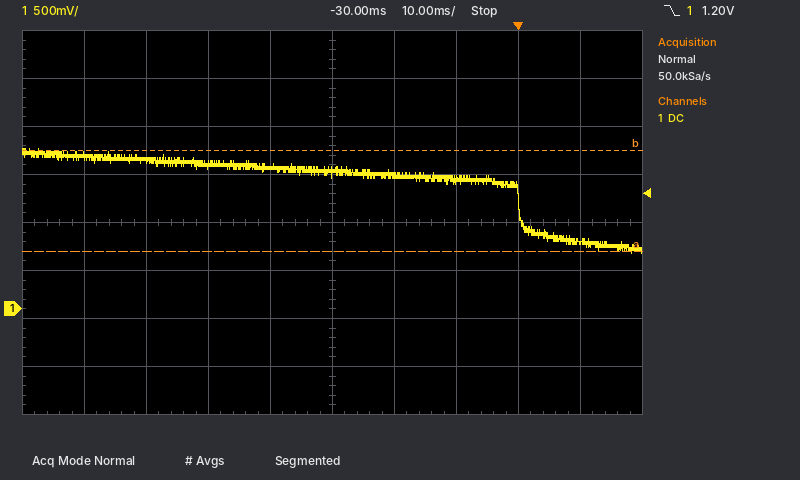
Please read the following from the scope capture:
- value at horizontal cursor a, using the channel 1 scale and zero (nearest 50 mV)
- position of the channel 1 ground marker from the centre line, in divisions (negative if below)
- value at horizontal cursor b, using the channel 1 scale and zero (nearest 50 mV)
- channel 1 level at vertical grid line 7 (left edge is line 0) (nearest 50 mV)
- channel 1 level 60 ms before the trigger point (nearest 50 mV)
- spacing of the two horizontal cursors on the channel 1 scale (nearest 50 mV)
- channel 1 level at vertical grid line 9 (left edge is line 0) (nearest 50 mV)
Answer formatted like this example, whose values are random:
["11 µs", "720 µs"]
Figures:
["600 mV", "-1.8 div", "1.65 V", "1.35 V", "1.55 V", "1.05 V", "700 mV"]
